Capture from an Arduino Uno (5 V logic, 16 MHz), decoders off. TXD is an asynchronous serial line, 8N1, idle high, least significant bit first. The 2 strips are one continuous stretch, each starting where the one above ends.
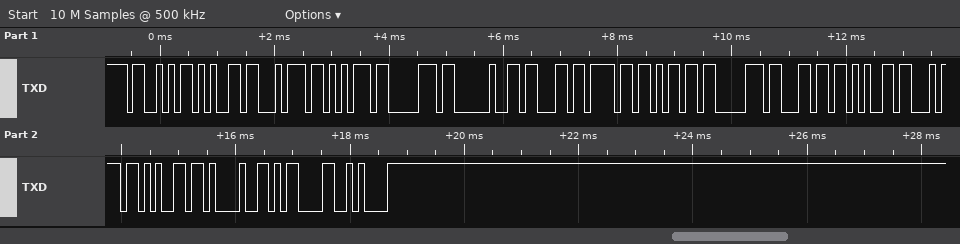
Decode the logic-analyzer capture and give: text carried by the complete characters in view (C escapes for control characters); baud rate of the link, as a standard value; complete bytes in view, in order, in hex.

"Setup complete!\r\n"
9600 baud
53 65 74 75 70 20 63 6F 6D 70 6C 65 74 65 21 0D 0A
